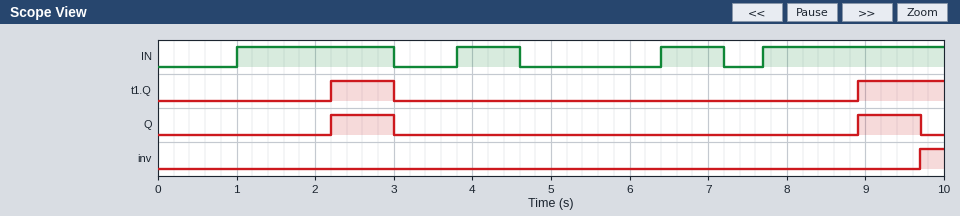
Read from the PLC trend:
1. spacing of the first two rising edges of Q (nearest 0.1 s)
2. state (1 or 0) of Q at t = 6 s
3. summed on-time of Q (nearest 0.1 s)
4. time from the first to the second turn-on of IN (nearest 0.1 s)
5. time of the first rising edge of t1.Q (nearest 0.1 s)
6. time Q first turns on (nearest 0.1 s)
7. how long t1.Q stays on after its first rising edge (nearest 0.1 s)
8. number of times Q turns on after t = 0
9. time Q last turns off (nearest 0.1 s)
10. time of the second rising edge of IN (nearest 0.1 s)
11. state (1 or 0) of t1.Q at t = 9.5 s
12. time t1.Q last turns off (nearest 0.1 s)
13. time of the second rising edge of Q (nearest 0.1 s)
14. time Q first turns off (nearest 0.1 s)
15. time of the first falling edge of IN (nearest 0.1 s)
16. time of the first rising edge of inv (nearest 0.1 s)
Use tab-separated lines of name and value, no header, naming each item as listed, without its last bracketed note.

spacing of the first two rising edges of Q	6.7 s
state (1 or 0) of Q at t = 6 s	0
summed on-time of Q	1.6 s
time from the first to the second turn-on of IN	2.8 s
time of the first rising edge of t1.Q	2.2 s
time Q first turns on	2.2 s
how long t1.Q stays on after its first rising edge	0.8 s
number of times Q turns on after t = 0	2
time Q last turns off	9.7 s
time of the second rising edge of IN	3.8 s
state (1 or 0) of t1.Q at t = 9.5 s	1
time t1.Q last turns off	3.0 s
time of the second rising edge of Q	8.9 s
time Q first turns off	3.0 s
time of the first falling edge of IN	3.0 s
time of the first rising edge of inv	9.7 s
